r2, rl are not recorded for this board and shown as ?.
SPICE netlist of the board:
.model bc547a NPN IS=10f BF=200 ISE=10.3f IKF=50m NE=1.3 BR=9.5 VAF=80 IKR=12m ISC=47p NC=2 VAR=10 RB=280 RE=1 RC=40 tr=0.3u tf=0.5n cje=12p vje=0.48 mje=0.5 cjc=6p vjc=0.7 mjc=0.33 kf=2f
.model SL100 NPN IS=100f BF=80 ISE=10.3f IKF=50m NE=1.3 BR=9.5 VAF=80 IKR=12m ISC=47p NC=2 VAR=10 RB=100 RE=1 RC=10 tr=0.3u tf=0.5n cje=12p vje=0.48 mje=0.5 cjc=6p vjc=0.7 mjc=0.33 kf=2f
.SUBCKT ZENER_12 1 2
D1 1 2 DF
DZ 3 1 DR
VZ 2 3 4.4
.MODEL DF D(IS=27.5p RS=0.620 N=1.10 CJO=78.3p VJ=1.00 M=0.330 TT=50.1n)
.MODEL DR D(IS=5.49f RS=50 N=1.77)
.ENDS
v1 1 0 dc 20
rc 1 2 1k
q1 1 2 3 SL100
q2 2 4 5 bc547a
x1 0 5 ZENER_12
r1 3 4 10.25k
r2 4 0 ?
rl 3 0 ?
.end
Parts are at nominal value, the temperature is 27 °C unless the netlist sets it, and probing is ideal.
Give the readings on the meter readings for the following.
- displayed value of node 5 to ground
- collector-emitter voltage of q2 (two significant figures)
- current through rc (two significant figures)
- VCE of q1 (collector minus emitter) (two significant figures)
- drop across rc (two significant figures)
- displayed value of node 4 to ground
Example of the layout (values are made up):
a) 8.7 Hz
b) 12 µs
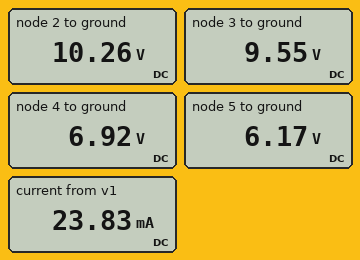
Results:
a) 6.17 V
b) 4.1 V
c) 9.7 mA
d) 10 V
e) 9.7 V
f) 6.92 V
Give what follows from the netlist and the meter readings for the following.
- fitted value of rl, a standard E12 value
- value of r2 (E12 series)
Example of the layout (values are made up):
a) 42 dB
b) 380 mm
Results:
a) 680 Ω
b) 39 kΩ
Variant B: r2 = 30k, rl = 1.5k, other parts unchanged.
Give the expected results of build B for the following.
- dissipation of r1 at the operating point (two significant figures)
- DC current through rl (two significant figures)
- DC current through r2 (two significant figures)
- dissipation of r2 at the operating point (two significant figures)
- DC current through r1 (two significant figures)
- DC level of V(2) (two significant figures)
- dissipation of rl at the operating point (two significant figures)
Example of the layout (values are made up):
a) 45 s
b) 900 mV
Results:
a) 960 µW
b) 6.7 mA
c) 230 µA
d) 1.6 mW
e) 310 µA
f) 11 V
g) 67 mW
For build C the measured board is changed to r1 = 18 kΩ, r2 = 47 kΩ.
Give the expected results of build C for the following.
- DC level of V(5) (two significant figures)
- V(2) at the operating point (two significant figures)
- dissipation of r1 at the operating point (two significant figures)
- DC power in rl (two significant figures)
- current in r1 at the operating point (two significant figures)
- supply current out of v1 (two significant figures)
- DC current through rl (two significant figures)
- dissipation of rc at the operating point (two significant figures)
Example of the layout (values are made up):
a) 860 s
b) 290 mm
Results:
a) 6.1 V
b) 11 V
c) 820 µW
d) 170 mW
e) 210 µA
f) 24 mA
g) 16 mA
h) 74 mW
